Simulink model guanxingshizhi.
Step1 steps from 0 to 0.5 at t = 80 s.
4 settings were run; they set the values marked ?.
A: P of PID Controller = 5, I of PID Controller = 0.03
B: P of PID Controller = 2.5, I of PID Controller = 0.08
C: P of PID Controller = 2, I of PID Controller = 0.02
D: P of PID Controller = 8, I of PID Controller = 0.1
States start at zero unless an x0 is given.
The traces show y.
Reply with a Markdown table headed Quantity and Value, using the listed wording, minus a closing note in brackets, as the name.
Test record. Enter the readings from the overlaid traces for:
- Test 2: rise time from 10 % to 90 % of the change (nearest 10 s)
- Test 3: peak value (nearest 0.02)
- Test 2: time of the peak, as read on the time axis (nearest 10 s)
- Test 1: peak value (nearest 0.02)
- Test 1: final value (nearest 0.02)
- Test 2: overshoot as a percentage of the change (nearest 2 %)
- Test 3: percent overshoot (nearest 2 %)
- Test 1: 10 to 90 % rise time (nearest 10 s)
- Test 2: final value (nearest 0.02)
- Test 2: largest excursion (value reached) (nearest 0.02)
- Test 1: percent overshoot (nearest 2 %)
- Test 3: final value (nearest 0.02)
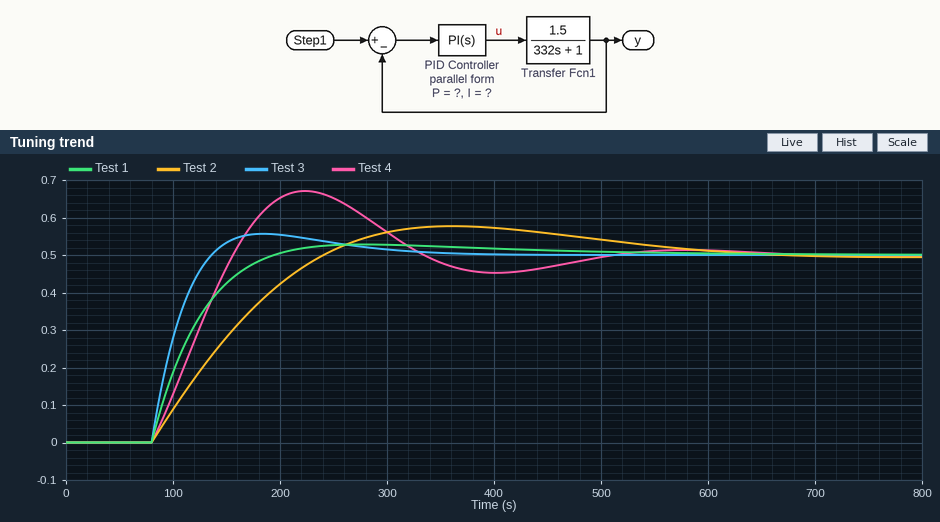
| Quantity | Value |
|---|---|
| Test 2: rise time from 10 % to 90 % of the change | 120 s |
| Test 3: peak value | 0.56 |
| Test 2: time of the peak, as read on the time axis | 360 s |
| Test 1: peak value | 0.52 |
| Test 1: final value | 0.50 |
| Test 2: overshoot as a percentage of the change | 16 % |
| Test 3: percent overshoot | 12 % |
| Test 1: 10 to 90 % rise time | 80 s |
| Test 2: final value | 0.50 |
| Test 2: largest excursion (value reached) | 0.58 |
| Test 1: percent overshoot | 6 % |
| Test 3: final value | 0.50 |
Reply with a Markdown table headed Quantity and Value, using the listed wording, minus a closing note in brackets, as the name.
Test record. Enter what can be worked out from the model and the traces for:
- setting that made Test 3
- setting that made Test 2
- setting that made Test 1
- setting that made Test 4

| Quantity | Value |
|---|---|
| setting that made Test 3 | D |
| setting that made Test 2 | C |
| setting that made Test 1 | A |
| setting that made Test 4 | B |
